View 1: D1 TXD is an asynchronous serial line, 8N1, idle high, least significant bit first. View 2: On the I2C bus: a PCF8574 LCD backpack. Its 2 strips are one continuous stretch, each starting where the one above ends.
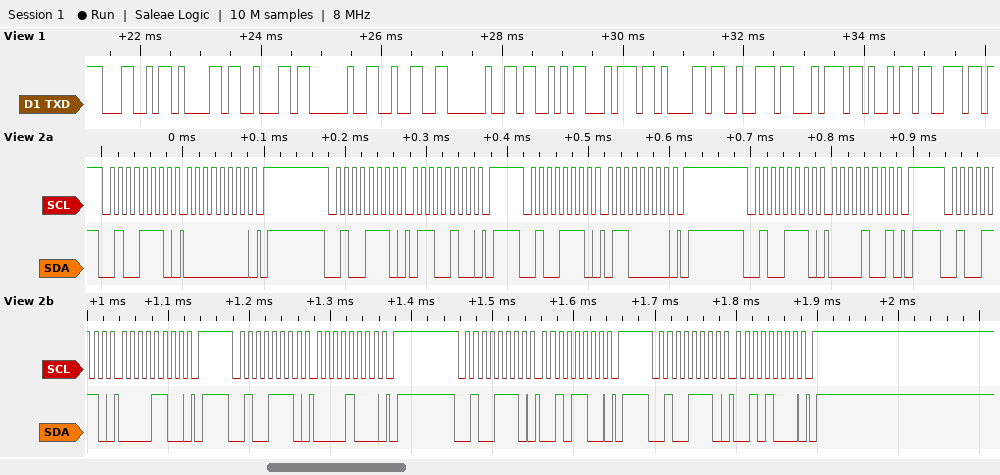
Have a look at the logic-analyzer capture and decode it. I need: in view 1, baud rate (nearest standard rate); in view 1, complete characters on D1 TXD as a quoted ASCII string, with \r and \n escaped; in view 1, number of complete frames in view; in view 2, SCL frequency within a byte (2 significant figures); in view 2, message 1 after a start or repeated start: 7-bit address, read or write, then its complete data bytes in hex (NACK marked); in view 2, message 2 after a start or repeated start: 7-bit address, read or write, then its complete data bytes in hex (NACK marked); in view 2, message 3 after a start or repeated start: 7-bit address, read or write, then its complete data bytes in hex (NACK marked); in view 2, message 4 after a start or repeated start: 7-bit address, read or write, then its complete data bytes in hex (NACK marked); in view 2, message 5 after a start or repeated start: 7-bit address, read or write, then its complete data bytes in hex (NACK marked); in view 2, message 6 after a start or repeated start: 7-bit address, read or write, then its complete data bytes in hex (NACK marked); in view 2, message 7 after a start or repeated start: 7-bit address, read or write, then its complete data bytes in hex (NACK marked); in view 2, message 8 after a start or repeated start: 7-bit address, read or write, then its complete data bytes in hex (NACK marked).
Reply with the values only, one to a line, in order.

9600 baud
"Lab 2 Startin"
13
100 kHz
0x27 write: 00
0x27 write: 64
0x27 write: 60
0x27 write: 09
0x27 write: 0C
0x27 write: 08
0x27 write: 2C
0x27 write: 28
